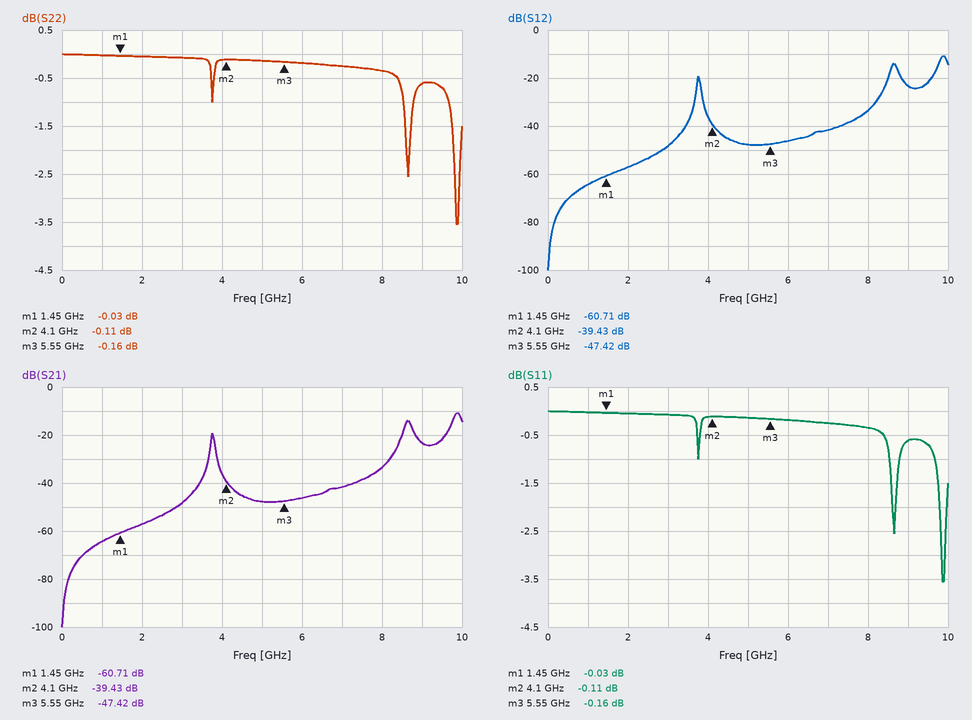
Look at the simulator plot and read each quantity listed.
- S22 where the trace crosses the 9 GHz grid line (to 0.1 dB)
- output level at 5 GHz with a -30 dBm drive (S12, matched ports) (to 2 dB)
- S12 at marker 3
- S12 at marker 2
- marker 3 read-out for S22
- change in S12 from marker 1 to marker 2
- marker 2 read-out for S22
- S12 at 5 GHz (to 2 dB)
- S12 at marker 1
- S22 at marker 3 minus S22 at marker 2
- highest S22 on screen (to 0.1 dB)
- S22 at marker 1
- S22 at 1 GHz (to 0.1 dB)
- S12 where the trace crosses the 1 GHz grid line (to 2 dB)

-0.6 dB
-78 dBm
-47.42 dB
-39.43 dB
-0.16 dB
21.28 dB
-0.11 dB
-48 dB
-60.71 dB
-0.05 dB
0.0 dB
-0.03 dB
0.0 dB
-64 dB
